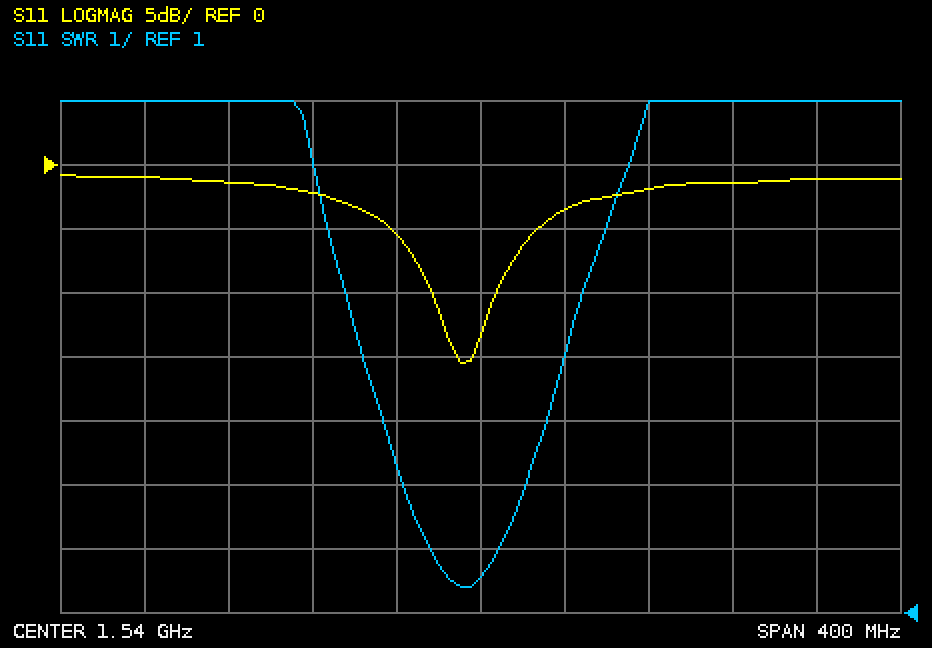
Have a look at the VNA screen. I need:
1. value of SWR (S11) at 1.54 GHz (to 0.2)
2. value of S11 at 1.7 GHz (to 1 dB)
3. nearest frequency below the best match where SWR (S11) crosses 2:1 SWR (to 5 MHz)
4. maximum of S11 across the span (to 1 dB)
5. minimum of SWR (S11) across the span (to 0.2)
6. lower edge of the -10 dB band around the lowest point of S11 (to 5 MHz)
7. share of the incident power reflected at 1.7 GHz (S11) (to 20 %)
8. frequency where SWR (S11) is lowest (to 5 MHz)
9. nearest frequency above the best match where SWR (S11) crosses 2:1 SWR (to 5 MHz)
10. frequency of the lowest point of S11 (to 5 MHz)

1.6
-1 dB
1.515 GHz
-1 dB
1.4
1.515 GHz
80 %
1.530 GHz
1.550 GHz
1.530 GHz
